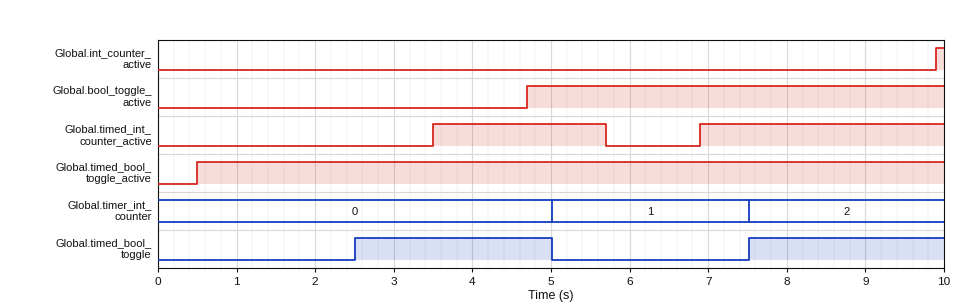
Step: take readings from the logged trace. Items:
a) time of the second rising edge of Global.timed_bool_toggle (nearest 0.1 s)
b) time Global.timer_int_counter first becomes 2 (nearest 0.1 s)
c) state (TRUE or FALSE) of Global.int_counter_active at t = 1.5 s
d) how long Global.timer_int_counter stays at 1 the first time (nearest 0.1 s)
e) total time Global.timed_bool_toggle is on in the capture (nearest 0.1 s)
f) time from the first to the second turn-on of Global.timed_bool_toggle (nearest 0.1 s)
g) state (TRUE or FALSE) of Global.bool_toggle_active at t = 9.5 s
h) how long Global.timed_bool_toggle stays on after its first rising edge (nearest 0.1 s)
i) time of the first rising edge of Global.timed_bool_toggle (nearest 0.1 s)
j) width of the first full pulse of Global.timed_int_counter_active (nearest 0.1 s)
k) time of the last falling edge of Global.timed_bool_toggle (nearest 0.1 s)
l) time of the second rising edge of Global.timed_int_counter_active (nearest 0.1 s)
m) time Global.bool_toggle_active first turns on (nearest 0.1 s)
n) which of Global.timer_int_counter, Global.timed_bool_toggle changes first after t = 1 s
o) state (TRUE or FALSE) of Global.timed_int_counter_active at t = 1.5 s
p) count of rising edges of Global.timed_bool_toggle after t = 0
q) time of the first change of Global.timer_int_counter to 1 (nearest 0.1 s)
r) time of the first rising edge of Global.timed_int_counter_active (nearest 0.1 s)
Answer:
7.5 s
7.5 s
FALSE
2.5 s
5.0 s
5.0 s
TRUE
2.5 s
2.5 s
2.2 s
5.0 s
6.9 s
4.7 s
Global.timed_bool_toggle
FALSE
2
5.0 s
3.5 s
